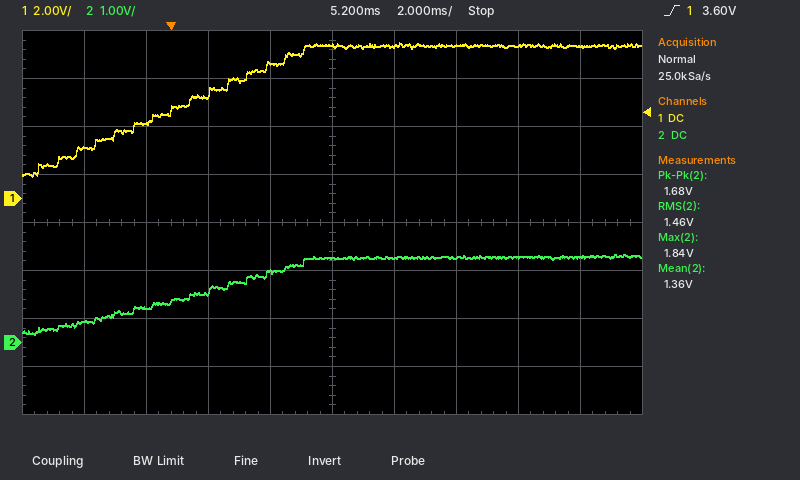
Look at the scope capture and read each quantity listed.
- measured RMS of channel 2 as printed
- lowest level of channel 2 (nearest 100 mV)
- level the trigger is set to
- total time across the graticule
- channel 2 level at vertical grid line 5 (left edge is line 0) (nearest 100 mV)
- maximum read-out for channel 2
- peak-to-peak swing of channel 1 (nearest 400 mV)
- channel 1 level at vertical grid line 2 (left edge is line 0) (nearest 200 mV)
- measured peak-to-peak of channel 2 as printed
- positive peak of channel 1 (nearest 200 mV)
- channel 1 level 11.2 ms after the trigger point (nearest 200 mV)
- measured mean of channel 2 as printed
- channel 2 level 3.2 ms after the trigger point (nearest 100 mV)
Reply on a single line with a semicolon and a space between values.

1.46 V; 200 mV; 3.60 V; 20 ms; 1.8 V; 1.84 V; 5.6 V; 3.2 V; 1.68 V; 6.4 V; 6.4 V; 1.36 V; 1.5 V
